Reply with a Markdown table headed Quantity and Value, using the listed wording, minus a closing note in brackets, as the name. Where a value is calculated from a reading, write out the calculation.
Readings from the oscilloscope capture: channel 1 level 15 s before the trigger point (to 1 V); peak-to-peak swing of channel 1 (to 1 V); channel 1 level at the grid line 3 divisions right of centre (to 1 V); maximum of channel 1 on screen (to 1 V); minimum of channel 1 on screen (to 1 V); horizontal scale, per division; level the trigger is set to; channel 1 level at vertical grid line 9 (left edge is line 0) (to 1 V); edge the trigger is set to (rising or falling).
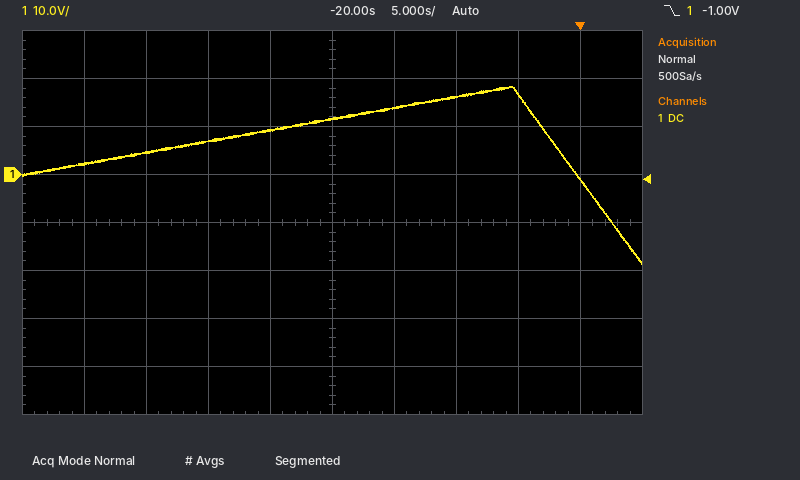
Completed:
| Quantity | Value |
|---|---|
| channel 1 level 15 s before the trigger point | 14 V |
| peak-to-peak swing of channel 1 | 18 V − (-19 V) = 37 V |
| channel 1 level at the grid line 3 divisions right of centre | 17 V |
| maximum of channel 1 on screen | 18 V |
| minimum of channel 1 on screen | -19 V |
| horizontal scale, per division | 5 s |
| level the trigger is set to | -1.00 V |
| channel 1 level at vertical grid line 9 (left edge is line 0) | -1 V |
| edge the trigger is set to | falling |
